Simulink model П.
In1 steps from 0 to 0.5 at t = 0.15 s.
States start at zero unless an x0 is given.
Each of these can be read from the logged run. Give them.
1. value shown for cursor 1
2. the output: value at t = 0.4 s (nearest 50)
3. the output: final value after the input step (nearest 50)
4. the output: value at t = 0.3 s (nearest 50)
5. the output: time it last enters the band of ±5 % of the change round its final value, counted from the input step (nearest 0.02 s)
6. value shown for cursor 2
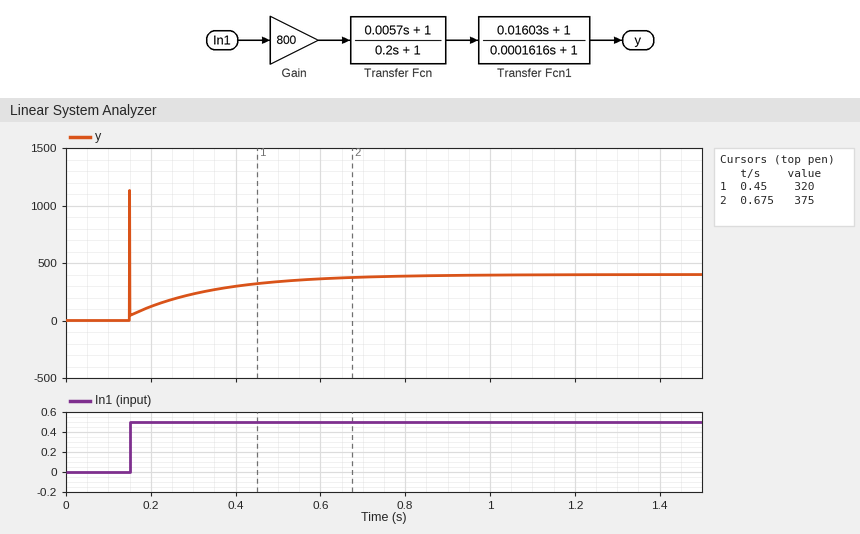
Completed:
320
300
400
250
0.58 s
375
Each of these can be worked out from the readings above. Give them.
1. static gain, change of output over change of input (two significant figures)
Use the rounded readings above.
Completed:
800
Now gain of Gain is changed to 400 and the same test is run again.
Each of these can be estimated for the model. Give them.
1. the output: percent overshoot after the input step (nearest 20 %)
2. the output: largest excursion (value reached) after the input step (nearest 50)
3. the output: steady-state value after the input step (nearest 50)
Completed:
180 %
550
200
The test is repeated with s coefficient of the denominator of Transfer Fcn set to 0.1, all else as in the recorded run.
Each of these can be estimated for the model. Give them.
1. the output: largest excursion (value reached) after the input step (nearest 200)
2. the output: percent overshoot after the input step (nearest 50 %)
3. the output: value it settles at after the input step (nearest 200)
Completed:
2200
450 %
400
